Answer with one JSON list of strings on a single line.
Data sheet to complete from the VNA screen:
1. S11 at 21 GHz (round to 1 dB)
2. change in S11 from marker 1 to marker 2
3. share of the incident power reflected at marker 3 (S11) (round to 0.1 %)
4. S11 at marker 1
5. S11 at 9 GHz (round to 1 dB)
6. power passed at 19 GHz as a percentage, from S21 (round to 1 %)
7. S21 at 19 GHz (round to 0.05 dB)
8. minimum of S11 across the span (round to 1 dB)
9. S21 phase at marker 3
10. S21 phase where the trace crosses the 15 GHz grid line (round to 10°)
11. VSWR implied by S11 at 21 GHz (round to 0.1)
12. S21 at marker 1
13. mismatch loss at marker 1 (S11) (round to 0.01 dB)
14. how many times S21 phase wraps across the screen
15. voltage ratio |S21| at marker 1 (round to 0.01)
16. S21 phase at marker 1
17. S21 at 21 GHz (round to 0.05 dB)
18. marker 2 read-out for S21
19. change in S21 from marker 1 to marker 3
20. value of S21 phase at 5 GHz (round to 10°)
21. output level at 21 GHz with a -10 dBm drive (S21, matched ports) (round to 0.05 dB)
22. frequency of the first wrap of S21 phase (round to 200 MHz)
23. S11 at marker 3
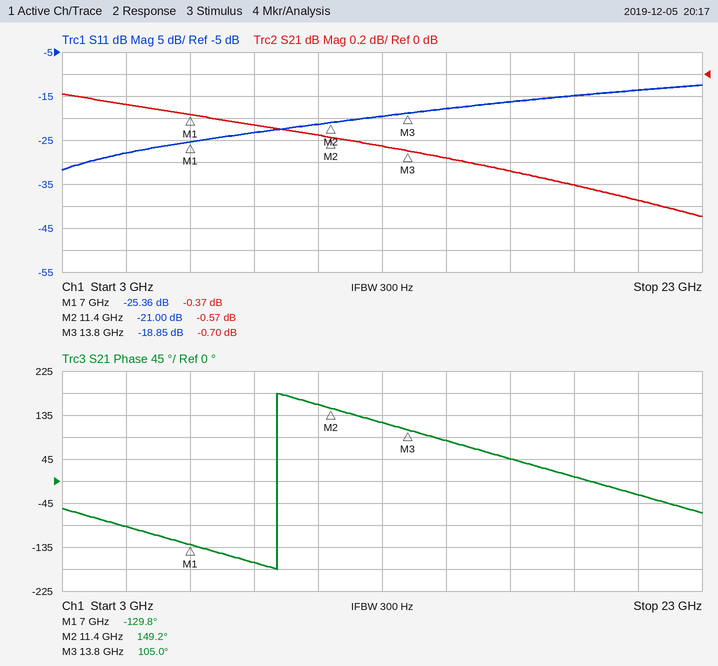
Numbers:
["-14 dB", "4.36 dB", "1.3 %", "-25.36 dB", "-23 dB", "79 %", "-1.00 dB", "-32 dB", "105.0°", "80°", "1.5", "-0.37 dB", "0.01 dB", "1", "0.96", "-129.8°", "-1.15 dB", "-0.57 dB", "-0.33 dB", "-90°", "-11.15 dBm", "9.8 GHz", "-18.85 dB"]
